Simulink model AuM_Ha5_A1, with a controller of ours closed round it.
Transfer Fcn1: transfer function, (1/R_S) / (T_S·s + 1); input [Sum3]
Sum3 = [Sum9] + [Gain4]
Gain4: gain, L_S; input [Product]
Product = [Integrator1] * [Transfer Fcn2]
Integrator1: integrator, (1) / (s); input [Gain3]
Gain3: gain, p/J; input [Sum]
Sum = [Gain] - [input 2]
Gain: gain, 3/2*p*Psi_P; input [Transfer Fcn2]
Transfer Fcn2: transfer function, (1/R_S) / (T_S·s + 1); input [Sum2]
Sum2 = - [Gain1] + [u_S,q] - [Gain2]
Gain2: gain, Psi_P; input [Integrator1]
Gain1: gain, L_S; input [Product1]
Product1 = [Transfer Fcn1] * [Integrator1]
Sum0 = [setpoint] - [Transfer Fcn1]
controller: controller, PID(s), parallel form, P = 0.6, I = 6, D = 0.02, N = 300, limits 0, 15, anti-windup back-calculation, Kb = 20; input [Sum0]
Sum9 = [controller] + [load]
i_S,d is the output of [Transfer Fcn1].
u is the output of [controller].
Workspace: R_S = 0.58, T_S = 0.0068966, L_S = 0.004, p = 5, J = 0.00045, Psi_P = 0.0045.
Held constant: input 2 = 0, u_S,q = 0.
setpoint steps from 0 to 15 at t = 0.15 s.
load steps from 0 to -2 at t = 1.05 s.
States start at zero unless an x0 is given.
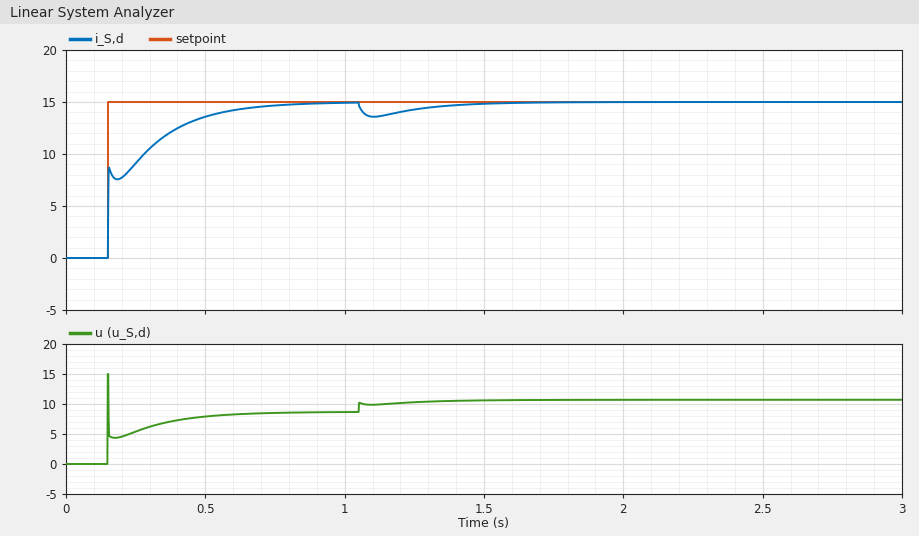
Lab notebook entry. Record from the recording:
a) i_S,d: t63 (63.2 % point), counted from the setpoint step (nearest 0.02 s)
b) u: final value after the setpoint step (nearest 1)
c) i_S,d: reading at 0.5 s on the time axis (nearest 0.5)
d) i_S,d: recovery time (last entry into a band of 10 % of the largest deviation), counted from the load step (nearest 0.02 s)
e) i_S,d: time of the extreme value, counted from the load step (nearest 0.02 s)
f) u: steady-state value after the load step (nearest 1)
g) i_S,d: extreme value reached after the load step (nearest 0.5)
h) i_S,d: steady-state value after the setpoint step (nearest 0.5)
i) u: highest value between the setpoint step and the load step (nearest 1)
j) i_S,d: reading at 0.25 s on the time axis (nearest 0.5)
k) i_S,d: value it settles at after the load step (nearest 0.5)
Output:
0.12 s
9
13.5
0.50 s
0.06 s
11
13.5
15.0
15
9.0
15.0
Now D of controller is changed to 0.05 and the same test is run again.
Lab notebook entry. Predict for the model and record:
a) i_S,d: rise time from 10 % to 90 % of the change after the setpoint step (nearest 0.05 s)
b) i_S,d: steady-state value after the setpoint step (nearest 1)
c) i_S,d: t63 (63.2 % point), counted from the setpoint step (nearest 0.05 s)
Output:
0.40 s
15
0.20 s
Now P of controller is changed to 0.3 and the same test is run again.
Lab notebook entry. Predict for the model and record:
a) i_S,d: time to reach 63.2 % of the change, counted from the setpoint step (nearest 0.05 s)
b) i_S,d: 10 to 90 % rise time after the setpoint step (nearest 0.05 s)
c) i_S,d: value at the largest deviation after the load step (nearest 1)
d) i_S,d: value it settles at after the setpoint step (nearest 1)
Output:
0.15 s
0.30 s
13
15
